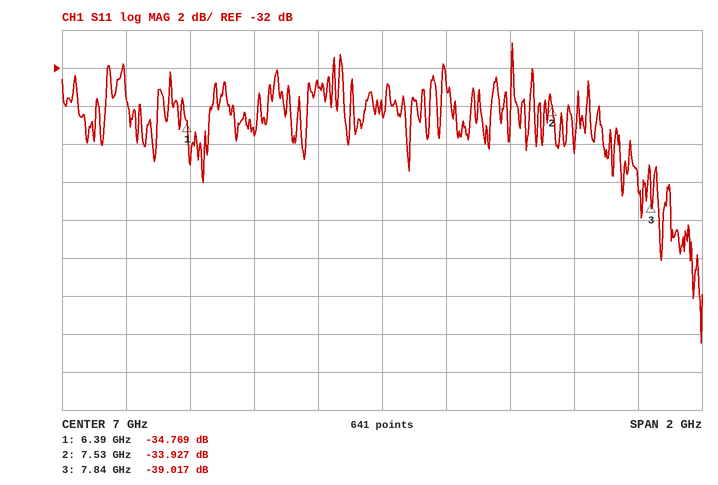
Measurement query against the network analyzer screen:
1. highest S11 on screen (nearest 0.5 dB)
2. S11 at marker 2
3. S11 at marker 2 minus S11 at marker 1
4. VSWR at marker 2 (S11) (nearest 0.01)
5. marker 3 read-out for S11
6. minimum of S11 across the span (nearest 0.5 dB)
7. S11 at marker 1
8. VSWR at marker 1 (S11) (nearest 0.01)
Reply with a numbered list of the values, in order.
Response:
1. -30.5 dB
2. -33.927 dB
3. 0.842 dB
4. 1.04
5. -39.017 dB
6. -46.5 dB
7. -34.769 dB
8. 1.04
